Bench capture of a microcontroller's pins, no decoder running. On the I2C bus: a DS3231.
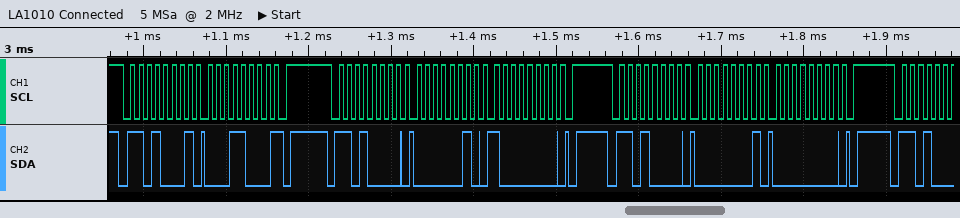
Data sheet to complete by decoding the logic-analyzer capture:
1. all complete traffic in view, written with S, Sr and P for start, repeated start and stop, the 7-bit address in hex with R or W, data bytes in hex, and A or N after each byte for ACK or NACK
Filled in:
S 68R A 18 N P S 68W A 02 A 80 A P S 68W A 01 A 00 A P
